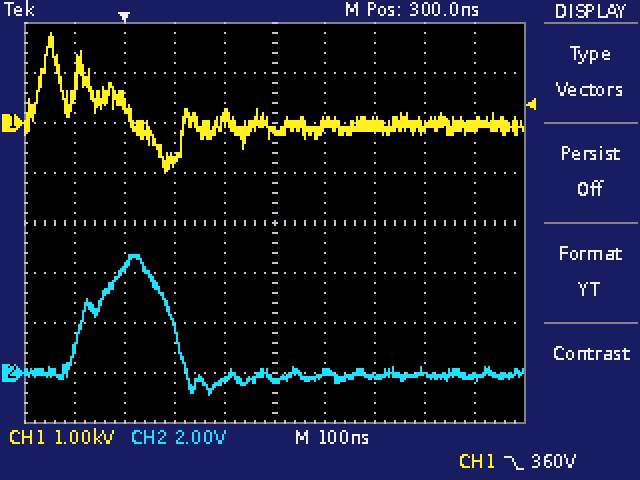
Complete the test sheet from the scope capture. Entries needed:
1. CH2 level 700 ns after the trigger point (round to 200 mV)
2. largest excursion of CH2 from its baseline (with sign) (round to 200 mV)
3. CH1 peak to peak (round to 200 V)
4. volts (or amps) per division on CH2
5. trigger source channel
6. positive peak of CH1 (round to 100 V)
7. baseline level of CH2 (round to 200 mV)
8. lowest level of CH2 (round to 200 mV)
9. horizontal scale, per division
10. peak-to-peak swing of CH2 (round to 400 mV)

-200 mV
+4.8 V
2.8 kV
2 V
CH1
1.8 kV
0.0 V
-800 mV
100 ns
5.6 V
